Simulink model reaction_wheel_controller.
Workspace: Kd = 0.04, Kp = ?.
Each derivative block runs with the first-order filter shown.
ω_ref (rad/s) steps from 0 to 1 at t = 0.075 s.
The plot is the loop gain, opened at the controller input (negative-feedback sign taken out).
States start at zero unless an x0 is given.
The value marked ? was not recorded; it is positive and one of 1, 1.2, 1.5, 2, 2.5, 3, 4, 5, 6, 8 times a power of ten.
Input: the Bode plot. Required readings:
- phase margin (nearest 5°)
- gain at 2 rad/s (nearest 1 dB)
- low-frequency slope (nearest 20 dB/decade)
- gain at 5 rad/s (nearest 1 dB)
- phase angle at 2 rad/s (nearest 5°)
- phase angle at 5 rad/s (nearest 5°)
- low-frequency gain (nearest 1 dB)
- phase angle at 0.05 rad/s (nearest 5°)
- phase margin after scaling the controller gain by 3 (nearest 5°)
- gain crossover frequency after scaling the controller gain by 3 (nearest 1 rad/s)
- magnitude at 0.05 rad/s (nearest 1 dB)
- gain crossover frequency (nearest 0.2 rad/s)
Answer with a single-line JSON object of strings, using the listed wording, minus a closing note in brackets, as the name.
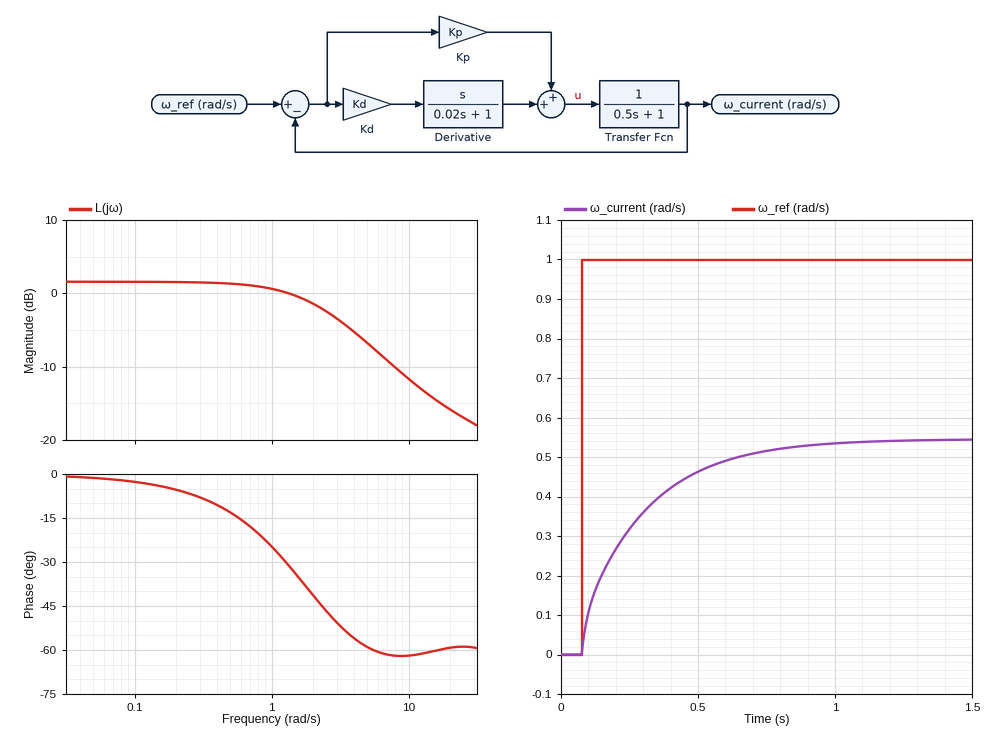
{"phase margin": "150°", "gain at 2 rad/s": "-1 dB", "low-frequency slope": "0 dB/decade", "gain at 5 rad/s": "-7 dB", "phase angle at 2 rad/s": "-40°", "phase angle at 5 rad/s": "-60°", "low-frequency gain": "2 dB", "phase angle at 0.05 rad/s": "0°", "phase margin after scaling the controller gain by 3": "120°", "gain crossover frequency after scaling the controller gain by 3": "7 rad/s", "magnitude at 0.05 rad/s": "2 dB", "gain crossover frequency": "1.4 rad/s"}
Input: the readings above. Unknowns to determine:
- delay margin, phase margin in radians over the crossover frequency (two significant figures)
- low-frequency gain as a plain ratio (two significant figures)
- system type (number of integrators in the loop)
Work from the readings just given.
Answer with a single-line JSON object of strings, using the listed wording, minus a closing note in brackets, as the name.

{"delay margin, phase margin in radians over the crossover frequency": "1.9 s", "low-frequency gain as a plain ratio": "1.3", "system type": "0"}
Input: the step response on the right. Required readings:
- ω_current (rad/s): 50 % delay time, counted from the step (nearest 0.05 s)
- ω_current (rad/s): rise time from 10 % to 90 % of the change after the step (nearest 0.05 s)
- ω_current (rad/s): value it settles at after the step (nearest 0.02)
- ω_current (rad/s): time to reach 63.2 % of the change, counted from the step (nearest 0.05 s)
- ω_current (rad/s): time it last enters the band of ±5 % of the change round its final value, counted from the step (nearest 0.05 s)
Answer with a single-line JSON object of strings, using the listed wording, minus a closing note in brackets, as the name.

{"ω_current (rad/s): 50 % delay time, counted from the step": "0.15 s", "ω_current (rad/s): rise time from 10 % to 90 % of the change after the step": "0.50 s", "ω_current (rad/s): value it settles at after the step": "0.54", "ω_current (rad/s): time to reach 63.2 % of the change, counted from the step": "0.20 s", "ω_current (rad/s): time it last enters the band of ±5 % of the change round its final value, counted from the step": "0.70 s"}
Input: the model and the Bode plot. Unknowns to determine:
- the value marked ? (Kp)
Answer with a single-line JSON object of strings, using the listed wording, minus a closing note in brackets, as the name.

{"the value marked ?": "1.2"}
